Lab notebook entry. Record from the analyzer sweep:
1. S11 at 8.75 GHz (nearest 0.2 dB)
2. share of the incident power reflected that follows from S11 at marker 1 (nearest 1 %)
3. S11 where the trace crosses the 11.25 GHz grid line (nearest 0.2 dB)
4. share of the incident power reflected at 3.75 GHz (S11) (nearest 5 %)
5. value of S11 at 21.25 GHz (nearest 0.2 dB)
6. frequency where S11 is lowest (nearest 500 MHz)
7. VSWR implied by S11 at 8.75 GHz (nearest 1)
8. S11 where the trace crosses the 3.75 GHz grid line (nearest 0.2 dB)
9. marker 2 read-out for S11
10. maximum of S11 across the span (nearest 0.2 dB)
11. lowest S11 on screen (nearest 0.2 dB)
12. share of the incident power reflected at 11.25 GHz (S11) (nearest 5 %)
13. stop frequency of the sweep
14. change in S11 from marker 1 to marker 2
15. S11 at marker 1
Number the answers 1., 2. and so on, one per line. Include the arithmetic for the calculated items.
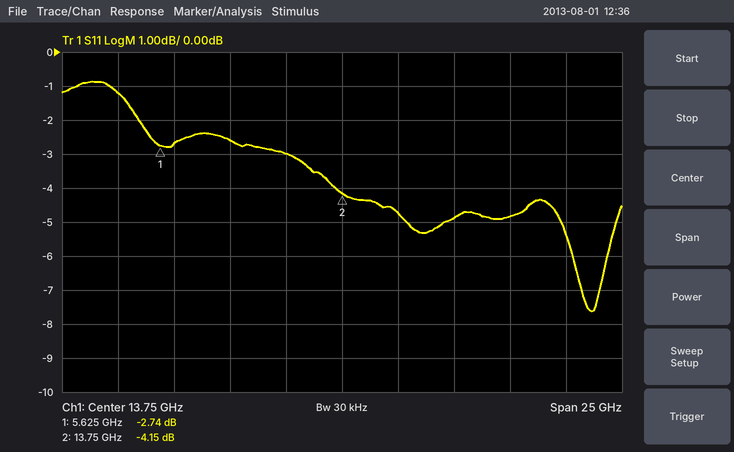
1. -2.6 dB
2. 10^(-2.74/10) ≈ 53 %
3. -3.0 dB
4. 10^(-1.2/10) ≈ 75.9 %, so 75 % to the nearest 5 %
5. -4.8 dB
6. 25.0 GHz
7. |Γ| = 10^(-2.6/20) = 0.7413; VSWR = (1 + 0.7413)/(1 − 0.7413) ≈ 7
8. -1.2 dB
9. -4.15 dB
10. -0.8 dB
11. -7.6 dB
12. 10^(-3/10) ≈ 50 %
13. 26.25 GHz
14. -4.15 − (-2.74) = -1.41 dB
15. -2.74 dB
